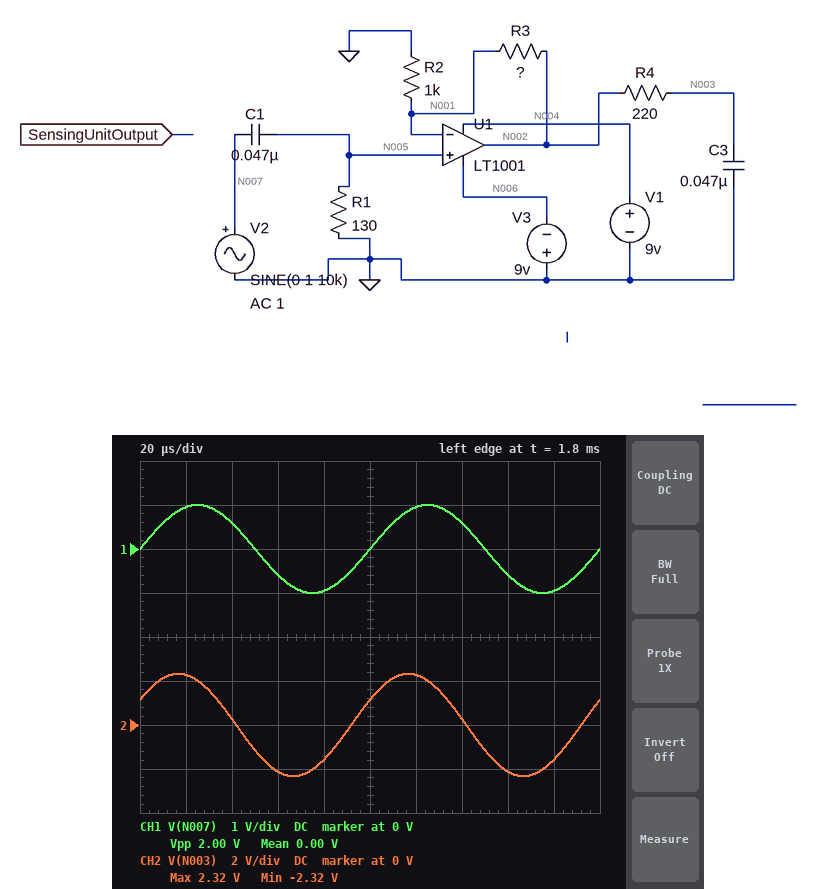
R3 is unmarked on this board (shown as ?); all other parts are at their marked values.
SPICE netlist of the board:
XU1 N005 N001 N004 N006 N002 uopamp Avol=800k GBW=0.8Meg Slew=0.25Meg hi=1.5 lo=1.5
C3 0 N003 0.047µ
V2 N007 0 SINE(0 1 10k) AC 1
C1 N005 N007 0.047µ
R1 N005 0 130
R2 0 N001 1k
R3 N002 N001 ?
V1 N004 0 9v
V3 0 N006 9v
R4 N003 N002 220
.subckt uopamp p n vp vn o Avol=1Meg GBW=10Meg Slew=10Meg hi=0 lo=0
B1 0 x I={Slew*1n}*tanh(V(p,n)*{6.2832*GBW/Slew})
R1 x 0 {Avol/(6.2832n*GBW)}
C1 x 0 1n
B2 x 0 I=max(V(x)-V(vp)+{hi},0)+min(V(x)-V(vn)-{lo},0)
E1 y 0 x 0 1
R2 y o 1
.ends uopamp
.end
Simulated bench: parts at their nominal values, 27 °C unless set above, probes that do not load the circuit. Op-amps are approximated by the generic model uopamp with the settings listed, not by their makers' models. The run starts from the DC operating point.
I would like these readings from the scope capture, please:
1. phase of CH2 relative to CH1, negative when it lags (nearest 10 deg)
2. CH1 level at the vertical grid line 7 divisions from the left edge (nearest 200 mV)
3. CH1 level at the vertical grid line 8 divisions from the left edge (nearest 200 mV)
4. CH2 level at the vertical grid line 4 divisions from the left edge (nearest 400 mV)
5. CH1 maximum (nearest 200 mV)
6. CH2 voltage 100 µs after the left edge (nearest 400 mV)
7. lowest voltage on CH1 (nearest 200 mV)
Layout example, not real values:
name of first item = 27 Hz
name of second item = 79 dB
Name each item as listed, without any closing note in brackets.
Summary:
phase of CH2 relative to CH1, negative when it lags = 30 deg
CH1 level at the vertical grid line 7 divisions from the left edge = 600 mV
CH1 level at the vertical grid line 8 divisions from the left edge = -600 mV
CH2 level at the vertical grid line 4 divisions from the left edge = -1.6 V
CH1 maximum = 1.0 V
CH2 voltage 100 µs after the left edge = 1.2 V
lowest voltage on CH1 = -1.0 V
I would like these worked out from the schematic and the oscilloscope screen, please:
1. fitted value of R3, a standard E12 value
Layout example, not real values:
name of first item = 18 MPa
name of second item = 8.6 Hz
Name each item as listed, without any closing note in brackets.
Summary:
fitted value of R3, a standard E12 value = 6.8 kΩ
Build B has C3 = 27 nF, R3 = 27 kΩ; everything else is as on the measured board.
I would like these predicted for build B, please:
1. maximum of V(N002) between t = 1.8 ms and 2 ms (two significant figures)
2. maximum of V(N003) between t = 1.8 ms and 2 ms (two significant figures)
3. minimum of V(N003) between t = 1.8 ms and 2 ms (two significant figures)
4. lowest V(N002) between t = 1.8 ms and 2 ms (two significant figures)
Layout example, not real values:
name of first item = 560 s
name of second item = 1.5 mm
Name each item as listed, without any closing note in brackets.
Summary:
maximum of V(N002) between t = 1.8 ms and 2 ms = 5.8 V
maximum of V(N003) between t = 1.8 ms and 2 ms = 5.1 V
minimum of V(N003) between t = 1.8 ms and 2 ms = -5.1 V
lowest V(N002) between t = 1.8 ms and 2 ms = -5.8 V
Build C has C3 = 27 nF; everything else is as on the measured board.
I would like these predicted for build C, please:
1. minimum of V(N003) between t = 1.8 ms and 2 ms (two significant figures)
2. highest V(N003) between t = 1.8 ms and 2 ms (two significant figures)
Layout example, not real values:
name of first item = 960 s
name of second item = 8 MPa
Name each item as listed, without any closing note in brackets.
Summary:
minimum of V(N003) between t = 1.8 ms and 2 ms = -2.6 V
highest V(N003) between t = 1.8 ms and 2 ms = 2.6 V
